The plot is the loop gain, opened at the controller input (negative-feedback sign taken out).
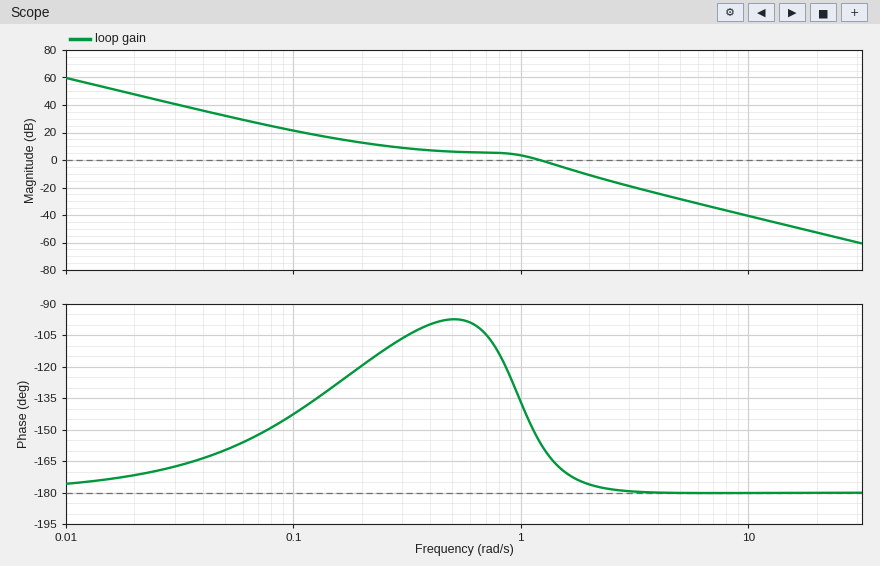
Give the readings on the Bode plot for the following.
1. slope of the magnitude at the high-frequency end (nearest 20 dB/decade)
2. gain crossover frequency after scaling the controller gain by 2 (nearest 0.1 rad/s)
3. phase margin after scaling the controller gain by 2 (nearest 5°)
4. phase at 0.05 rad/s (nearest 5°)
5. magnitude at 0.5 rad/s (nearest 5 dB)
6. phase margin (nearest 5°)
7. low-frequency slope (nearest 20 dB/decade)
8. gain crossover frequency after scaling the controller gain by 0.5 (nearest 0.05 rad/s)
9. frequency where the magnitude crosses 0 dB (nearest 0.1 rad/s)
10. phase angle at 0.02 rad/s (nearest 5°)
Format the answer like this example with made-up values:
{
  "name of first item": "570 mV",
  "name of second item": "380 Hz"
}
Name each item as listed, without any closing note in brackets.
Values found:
{
  "slope of the magnitude at the high-frequency end": "-40 dB/decade",
  "gain crossover frequency after scaling the controller gain by 2": "1.6 rad/s",
  "phase margin after scaling the controller gain by 2": "10°",
  "phase at 0.05 rad/s": "-160°",
  "magnitude at 0.5 rad/s": "5 dB",
  "phase margin": "25°",
  "low-frequency slope": "-40 dB/decade",
  "gain crossover frequency after scaling the controller gain by 0.5": "0.50 rad/s",
  "frequency where the magnitude crosses 0 dB": "1.2 rad/s",
  "phase angle at 0.02 rad/s": "-170°"
}
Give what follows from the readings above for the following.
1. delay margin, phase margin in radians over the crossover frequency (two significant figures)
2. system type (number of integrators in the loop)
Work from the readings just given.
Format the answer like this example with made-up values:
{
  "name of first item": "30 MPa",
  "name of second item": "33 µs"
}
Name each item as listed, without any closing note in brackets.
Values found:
{
  "delay margin, phase margin in radians over the crossover frequency": "0.36 s",
  "system type": "2"
}
